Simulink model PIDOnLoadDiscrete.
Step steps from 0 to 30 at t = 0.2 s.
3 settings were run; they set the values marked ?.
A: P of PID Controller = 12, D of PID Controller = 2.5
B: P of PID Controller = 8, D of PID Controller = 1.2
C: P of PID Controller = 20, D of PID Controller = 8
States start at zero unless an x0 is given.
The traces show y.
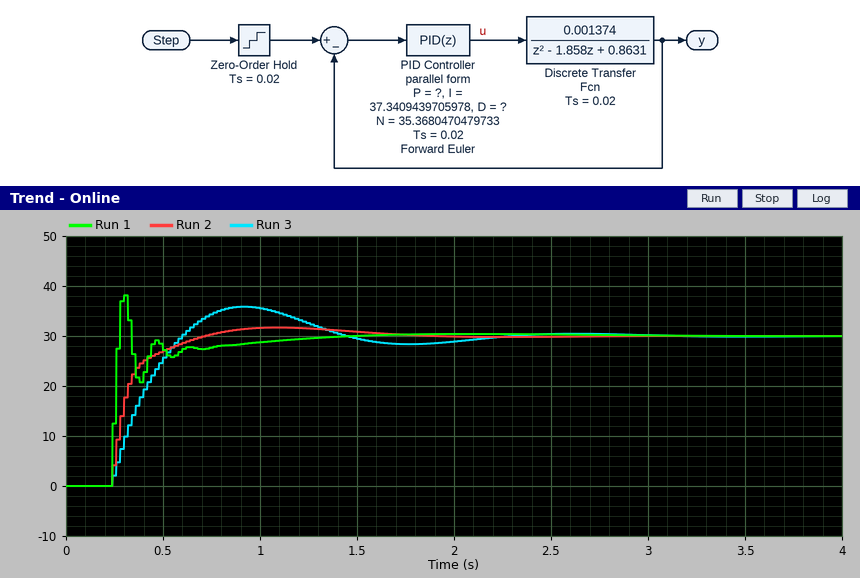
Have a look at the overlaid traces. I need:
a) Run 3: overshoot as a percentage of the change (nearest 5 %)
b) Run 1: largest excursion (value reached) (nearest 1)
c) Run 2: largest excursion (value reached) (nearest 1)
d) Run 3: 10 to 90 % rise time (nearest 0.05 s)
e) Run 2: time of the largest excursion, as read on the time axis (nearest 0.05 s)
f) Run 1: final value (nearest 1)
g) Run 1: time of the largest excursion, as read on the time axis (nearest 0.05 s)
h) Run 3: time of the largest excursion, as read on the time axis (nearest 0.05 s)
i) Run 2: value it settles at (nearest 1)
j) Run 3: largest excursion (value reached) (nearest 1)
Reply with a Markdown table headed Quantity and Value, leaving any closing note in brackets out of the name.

| Quantity | Value |
|---|---|
| Run 3: overshoot as a percentage of the change | 20 % |
| Run 1: largest excursion (value reached) | 38 |
| Run 2: largest excursion (value reached) | 32 |
| Run 3: 10 to 90 % rise time | 0.30 s |
| Run 2: time of the largest excursion, as read on the time axis | 1.10 s |
| Run 1: final value | 30 |
| Run 1: time of the largest excursion, as read on the time axis | 0.30 s |
| Run 3: time of the largest excursion, as read on the time axis | 0.90 s |
| Run 2: value it settles at | 30 |
| Run 3: largest excursion (value reached) | 36 |
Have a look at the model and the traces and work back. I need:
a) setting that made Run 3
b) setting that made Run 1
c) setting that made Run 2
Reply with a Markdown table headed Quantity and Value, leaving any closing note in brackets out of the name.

| Quantity | Value |
|---|---|
| setting that made Run 3 | B |
| setting that made Run 1 | C |
| setting that made Run 2 | A |
